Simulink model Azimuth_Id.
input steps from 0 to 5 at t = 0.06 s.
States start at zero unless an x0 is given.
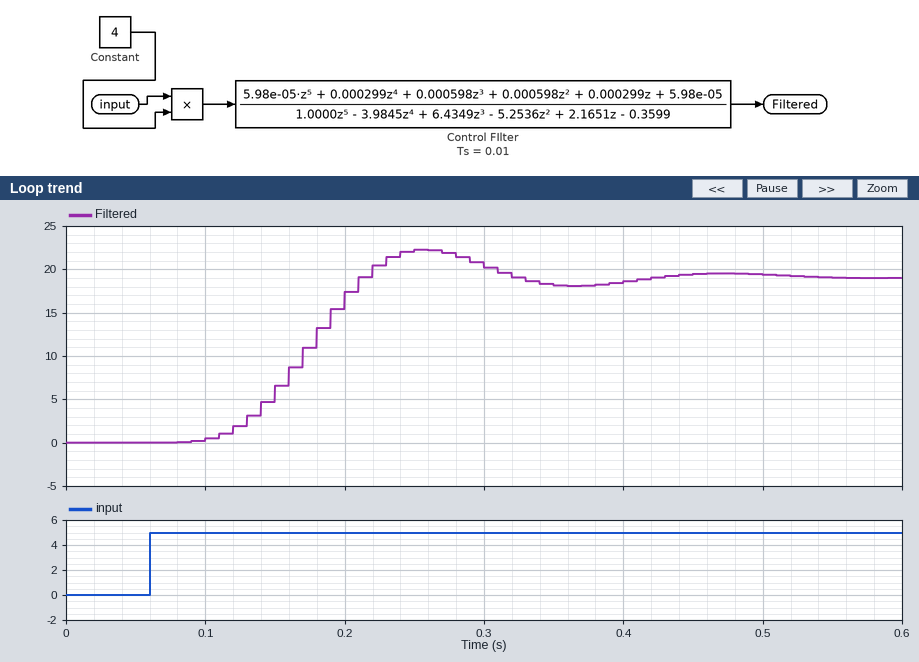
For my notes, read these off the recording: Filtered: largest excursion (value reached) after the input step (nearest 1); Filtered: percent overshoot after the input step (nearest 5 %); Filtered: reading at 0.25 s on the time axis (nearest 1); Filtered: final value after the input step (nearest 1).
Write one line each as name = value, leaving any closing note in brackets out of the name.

Filtered: largest excursion (value reached) after the input step = 22
Filtered: percent overshoot after the input step = 15 %
Filtered: reading at 0.25 s on the time axis = 22
Filtered: final value after the input step = 19
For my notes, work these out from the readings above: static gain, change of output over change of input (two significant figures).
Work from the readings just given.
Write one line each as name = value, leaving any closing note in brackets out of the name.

static gain, change of output over change of input = 3.8
